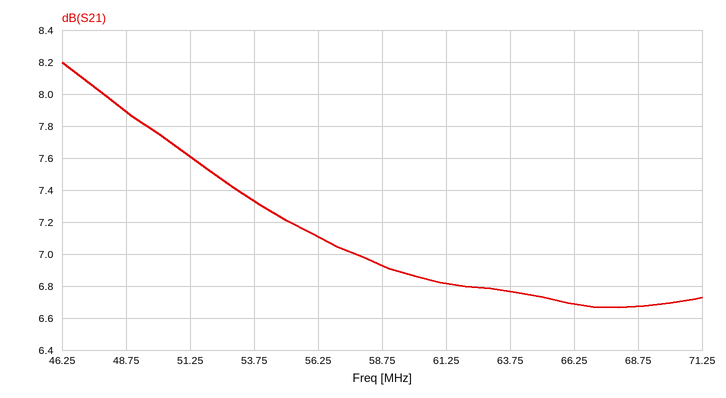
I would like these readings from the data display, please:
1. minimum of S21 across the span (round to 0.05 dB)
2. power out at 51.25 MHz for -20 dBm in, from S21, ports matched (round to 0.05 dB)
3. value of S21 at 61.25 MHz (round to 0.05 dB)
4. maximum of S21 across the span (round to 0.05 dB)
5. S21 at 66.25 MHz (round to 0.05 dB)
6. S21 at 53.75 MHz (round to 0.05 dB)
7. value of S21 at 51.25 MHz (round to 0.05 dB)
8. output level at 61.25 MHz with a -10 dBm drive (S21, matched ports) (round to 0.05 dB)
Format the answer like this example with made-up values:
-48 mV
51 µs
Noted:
6.65 dB
-12.40 dBm
6.80 dB
8.20 dB
6.70 dB
7.35 dB
7.60 dB
-3.20 dBm
